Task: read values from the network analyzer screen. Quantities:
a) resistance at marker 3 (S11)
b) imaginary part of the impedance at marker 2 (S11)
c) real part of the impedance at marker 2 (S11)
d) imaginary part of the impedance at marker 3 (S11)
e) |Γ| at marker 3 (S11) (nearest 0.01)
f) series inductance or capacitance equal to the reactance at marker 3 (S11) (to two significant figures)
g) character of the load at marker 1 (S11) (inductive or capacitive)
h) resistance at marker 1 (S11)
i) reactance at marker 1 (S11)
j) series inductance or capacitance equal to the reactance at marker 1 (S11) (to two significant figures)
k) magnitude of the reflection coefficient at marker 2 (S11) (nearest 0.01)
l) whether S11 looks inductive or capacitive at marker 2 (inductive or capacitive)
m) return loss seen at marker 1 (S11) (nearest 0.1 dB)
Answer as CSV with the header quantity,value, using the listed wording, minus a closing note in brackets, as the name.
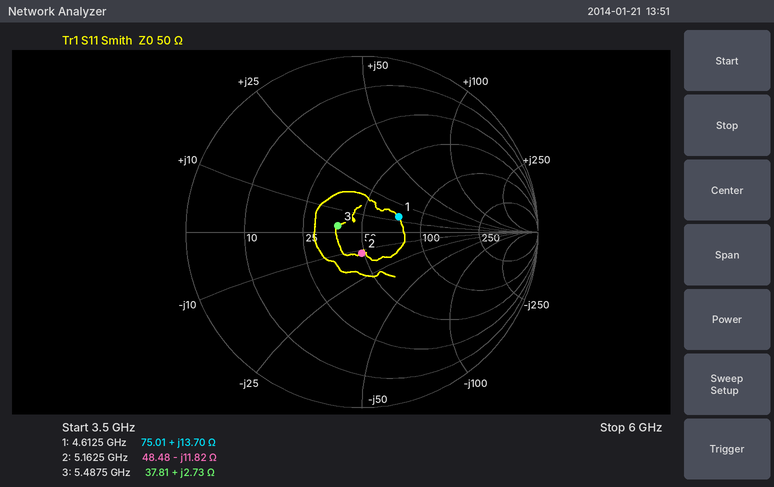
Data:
quantity,value
resistance at marker 3,37.81 Ω
imaginary part of the impedance at marker 2,-11.82 Ω
real part of the impedance at marker 2,48.48 Ω
imaginary part of the impedance at marker 3,+2.73 Ω
|Γ| at marker 3 (S11),0.14
series inductance or capacitance equal to the reactance at marker 3 (S11),79 pH
character of the load at marker 1 (S11),inductive
resistance at marker 1,75.01 Ω
reactance at marker 1,+13.70 Ω
series inductance or capacitance equal to the reactance at marker 1 (S11),470 pH
magnitude of the reflection coefficient at marker 2 (S11),0.12
whether S11 looks inductive or capacitive at marker 2,capacitive
return loss seen at marker 1 (S11),12.9 dB
